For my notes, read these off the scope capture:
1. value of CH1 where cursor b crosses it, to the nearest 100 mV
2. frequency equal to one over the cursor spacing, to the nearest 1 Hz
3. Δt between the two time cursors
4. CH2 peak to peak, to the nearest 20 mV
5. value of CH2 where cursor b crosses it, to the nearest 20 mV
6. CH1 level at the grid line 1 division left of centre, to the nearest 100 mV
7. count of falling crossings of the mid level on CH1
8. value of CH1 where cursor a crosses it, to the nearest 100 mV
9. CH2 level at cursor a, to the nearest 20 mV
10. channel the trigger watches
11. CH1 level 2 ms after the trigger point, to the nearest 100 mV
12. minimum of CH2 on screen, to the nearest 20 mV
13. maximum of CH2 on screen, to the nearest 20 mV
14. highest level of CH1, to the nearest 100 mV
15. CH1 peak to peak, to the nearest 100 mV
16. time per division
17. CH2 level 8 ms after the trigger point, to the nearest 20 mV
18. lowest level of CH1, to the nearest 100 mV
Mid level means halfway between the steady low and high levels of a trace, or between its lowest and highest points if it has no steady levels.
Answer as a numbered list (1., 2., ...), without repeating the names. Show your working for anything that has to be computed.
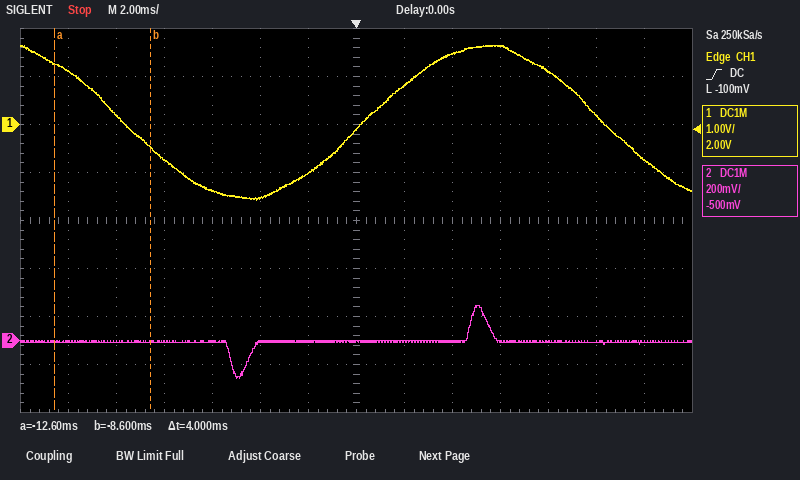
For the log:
1. -500 mV
2. 1 / 4 ms ≈ 250 Hz
3. 4 ms
4. 140 mV − (-160 mV) = 300 mV
5. 0 mV
6. -1.0 V
7. 2
8. 1.3 V
9. 0 mV
10. CH1
11. 800 mV
12. -160 mV
13. 140 mV
14. 1.6 V
15. 1.6 V − (-1.6 V) = 3.2 V
16. 2 ms
17. 0 mV
18. -1.6 V
